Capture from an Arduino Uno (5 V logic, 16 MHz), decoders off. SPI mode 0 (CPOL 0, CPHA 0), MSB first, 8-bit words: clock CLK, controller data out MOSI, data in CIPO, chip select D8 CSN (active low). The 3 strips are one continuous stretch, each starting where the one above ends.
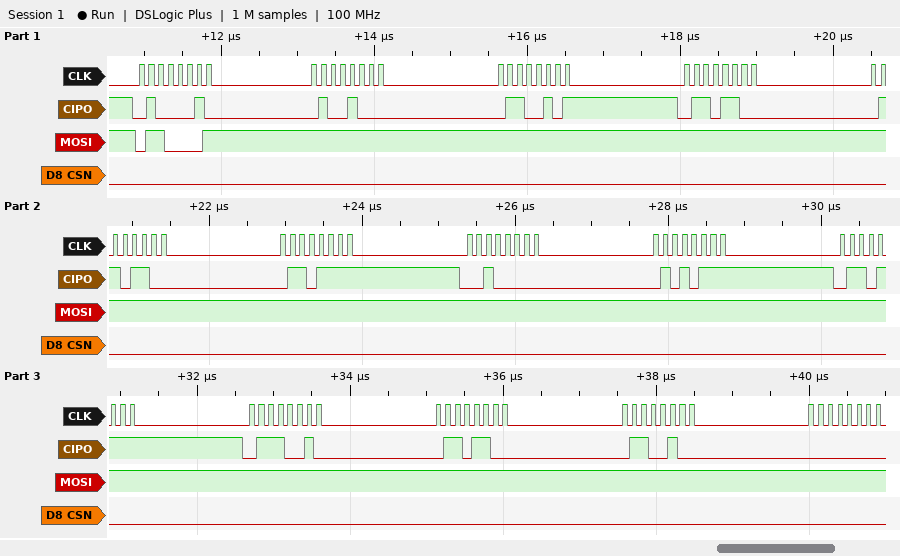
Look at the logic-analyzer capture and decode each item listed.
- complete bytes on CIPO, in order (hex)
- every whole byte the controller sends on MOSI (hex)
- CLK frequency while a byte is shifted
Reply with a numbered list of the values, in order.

1. 42 48 65 6C 6C 6F 20 57 6F 72 6C 64 00
2. 61 FF FF FF FF FF FF FF FF FF FF FF FF
3. 8 MHz
